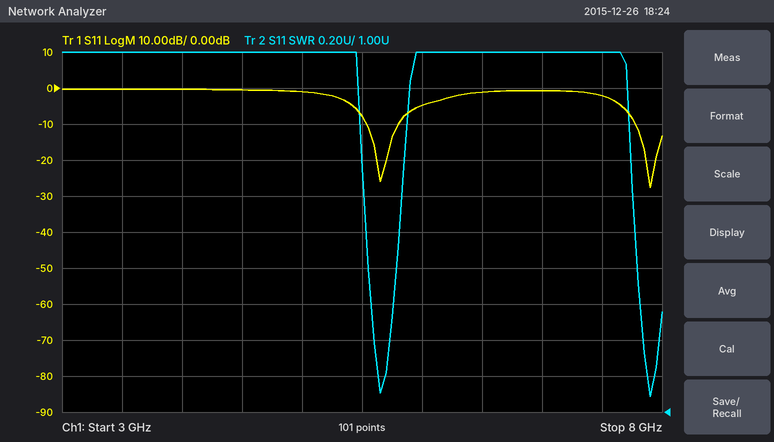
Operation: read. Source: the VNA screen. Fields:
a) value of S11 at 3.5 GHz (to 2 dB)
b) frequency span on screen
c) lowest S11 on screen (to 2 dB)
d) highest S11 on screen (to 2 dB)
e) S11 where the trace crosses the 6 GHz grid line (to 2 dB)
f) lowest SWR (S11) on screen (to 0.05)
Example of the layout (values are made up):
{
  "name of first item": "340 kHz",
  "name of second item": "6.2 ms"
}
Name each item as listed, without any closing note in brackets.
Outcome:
{
  "value of S11 at 3.5 GHz": "0 dB",
  "frequency span on screen": "5 GHz",
  "lowest S11 on screen": "-28 dB",
  "highest S11 on screen": "0 dB",
  "S11 where the trace crosses the 6 GHz grid line": "-4 dB",
  "lowest SWR (S11) on screen": "1.10"
}
